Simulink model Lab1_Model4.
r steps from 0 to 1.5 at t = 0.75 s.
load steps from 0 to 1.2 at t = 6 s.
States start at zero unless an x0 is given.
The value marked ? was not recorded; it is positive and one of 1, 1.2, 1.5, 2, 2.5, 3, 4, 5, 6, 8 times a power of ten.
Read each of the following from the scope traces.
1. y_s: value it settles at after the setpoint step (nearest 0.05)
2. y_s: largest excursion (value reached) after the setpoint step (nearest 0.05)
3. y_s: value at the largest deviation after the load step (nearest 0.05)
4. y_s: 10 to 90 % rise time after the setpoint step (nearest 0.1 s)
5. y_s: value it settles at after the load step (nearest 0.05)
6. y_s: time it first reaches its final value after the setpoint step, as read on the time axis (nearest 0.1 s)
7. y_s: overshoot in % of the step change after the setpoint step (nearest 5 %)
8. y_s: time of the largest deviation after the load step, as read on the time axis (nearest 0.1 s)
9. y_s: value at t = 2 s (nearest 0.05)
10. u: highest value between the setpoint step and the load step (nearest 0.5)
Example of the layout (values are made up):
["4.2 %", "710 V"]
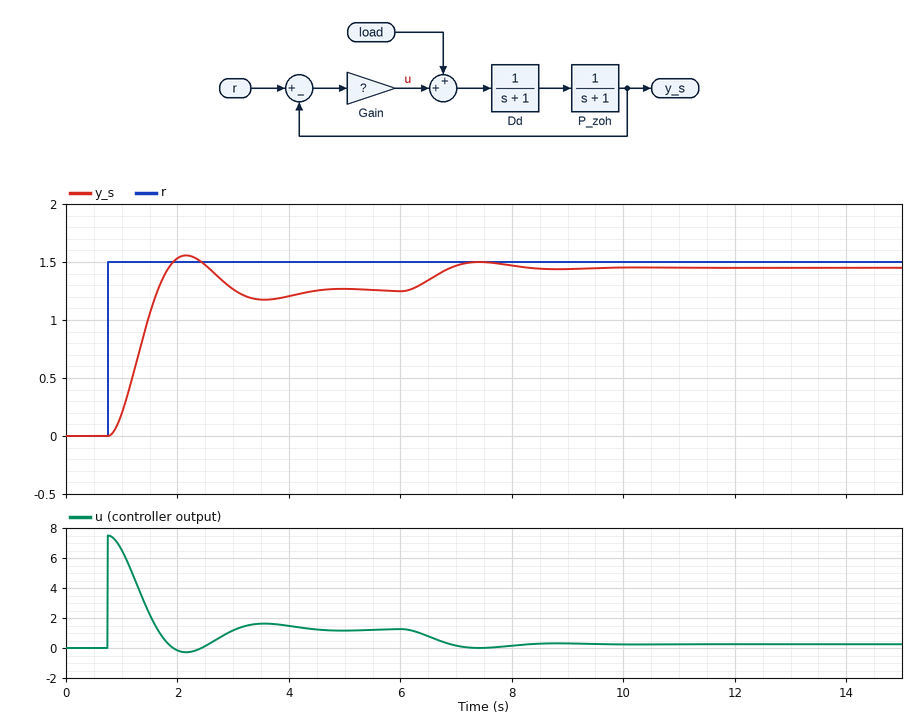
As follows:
["1.25", "1.55", "1.50", "0.6 s", "1.45", "1.6 s", "25 %", "7.4 s", "1.55", "7.5"]
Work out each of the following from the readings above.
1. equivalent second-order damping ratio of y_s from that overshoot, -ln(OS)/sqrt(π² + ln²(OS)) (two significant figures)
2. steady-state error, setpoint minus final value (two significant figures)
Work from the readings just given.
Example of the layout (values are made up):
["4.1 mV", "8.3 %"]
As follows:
["0.40", "0.25"]
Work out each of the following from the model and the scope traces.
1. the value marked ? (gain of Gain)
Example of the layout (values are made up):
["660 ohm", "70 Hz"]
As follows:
["5"]
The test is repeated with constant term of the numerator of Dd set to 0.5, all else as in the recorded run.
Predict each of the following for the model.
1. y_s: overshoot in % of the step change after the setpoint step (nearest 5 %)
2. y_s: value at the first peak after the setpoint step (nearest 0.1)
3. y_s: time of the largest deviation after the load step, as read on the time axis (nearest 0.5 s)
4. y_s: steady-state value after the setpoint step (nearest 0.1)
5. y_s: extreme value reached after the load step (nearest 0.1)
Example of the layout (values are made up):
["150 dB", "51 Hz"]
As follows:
["15 %", "1.2", "8.0 s", "1.1", "1.3"]
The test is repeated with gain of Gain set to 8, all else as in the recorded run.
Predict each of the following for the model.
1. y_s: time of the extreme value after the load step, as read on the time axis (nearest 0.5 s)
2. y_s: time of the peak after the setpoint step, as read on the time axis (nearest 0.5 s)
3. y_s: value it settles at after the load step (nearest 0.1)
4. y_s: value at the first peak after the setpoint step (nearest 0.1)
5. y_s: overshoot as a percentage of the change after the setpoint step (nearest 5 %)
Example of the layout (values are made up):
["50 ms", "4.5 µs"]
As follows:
["7.0 s", "2.0 s", "1.5", "1.8", "35 %"]
